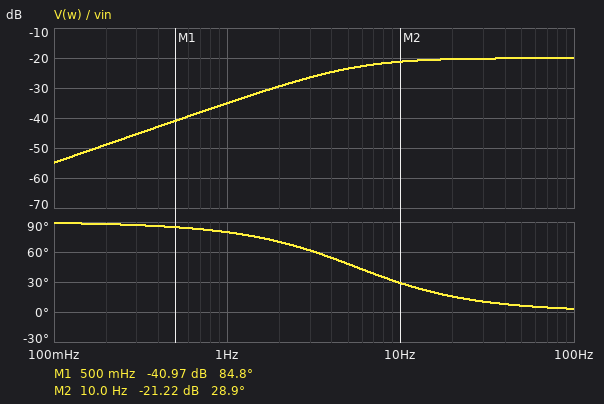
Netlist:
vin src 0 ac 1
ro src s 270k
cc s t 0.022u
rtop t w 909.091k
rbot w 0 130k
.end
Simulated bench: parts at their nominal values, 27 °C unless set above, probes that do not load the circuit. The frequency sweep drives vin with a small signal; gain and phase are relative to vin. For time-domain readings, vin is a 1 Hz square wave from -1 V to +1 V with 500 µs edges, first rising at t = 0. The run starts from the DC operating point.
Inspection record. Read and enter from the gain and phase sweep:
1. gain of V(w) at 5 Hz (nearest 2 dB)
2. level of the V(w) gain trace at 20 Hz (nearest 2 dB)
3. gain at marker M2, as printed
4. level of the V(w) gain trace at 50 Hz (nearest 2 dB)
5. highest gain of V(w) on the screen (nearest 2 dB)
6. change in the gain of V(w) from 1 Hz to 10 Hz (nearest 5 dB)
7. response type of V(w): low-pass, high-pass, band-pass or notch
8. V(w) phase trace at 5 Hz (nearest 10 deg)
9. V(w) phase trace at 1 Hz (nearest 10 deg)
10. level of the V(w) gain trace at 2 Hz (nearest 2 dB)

-24 dB
-20 dB
-21.22 dB
-20 dB
-20 dB
15 dB
high-pass
50 deg
80 deg
-30 dB
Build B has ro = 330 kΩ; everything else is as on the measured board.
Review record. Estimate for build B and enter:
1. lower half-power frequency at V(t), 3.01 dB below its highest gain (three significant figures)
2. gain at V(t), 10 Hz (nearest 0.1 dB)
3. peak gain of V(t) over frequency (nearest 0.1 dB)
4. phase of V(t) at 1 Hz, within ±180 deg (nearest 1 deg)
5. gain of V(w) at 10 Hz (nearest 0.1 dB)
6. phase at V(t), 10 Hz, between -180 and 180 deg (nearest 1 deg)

5.28 Hz
-3.5 dB
-2.4 dB
79 deg
-21.5 dB
28 deg
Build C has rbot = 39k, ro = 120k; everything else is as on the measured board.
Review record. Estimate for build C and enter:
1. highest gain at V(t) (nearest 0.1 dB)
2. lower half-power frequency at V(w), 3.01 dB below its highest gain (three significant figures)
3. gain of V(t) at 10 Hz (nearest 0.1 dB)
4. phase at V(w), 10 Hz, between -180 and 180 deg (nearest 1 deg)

-1.0 dB
6.77 Hz
-2.7 dB
34 deg
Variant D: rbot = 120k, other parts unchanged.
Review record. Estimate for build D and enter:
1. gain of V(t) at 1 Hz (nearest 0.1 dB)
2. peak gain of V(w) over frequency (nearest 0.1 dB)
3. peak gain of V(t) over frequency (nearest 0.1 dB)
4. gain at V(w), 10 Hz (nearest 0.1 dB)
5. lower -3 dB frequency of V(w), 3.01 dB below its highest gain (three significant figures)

-17.1 dB
-20.7 dB
-2.0 dB
-21.9 dB
5.57 Hz
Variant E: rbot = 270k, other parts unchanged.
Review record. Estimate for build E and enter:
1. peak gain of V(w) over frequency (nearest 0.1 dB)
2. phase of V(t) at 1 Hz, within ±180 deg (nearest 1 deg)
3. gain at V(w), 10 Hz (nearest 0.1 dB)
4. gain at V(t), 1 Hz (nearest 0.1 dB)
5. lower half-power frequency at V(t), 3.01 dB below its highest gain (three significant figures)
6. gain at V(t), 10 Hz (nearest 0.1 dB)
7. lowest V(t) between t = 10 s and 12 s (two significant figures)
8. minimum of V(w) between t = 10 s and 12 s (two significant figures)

-14.6 dB
79 deg
-15.6 dB
-15.9 dB
4.99 Hz
-2.8 dB
-1.6 V
-370 mV
